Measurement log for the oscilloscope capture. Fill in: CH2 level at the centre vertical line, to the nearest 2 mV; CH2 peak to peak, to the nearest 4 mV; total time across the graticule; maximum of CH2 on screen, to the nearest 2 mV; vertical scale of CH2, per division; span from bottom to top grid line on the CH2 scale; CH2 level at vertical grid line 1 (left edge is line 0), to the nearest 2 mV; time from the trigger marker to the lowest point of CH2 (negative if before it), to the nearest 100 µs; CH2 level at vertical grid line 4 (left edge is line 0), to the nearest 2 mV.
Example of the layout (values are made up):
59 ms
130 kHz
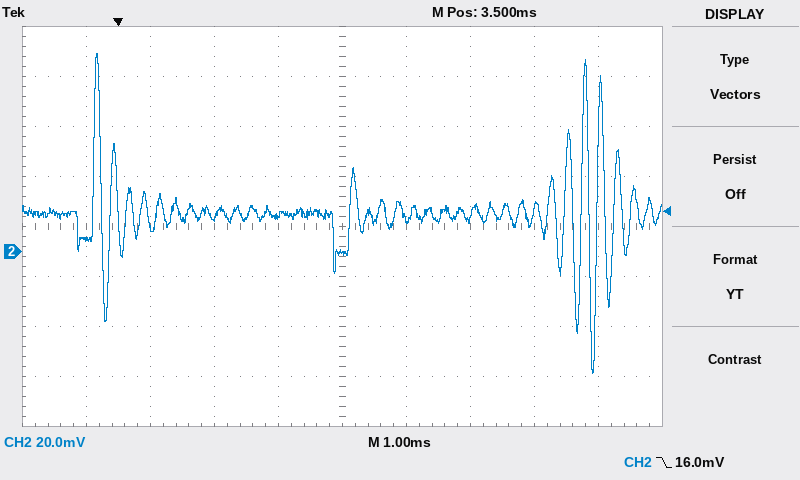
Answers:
0 mV
128 mV
10 ms
80 mV
20 mV
160 mV
4 mV
+7.4 ms
14 mV
